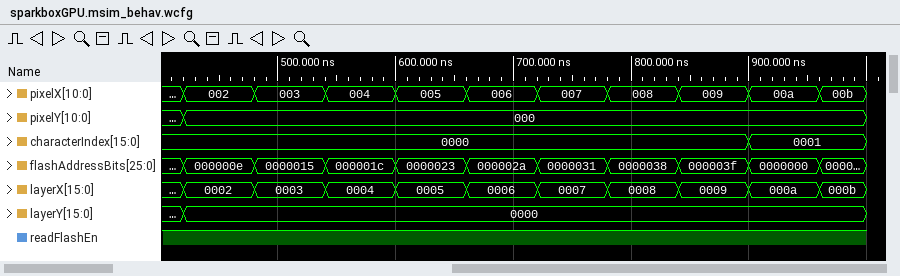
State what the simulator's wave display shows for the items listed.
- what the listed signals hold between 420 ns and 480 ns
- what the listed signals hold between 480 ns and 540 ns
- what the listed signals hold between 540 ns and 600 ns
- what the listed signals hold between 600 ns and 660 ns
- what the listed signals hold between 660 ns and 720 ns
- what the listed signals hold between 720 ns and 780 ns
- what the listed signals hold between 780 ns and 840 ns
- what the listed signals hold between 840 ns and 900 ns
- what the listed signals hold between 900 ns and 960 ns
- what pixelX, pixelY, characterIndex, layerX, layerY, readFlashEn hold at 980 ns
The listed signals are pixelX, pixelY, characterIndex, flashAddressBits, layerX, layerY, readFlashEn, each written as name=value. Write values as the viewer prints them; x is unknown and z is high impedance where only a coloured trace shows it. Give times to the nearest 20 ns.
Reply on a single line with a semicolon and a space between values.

pixelX=002, pixelY=000, characterIndex=0000, flashAddressBits=000000e, layerX=0002, layerY=0000, readFlashEn=1; pixelX=003, pixelY=000, characterIndex=0000, flashAddressBits=0000015, layerX=0003, layerY=0000, readFlashEn=1; pixelX=004, pixelY=000, characterIndex=0000, flashAddressBits=000001c, layerX=0004, layerY=0000, readFlashEn=1; pixelX=005, pixelY=000, characterIndex=0000, flashAddressBits=0000023, layerX=0005, layerY=0000, readFlashEn=1; pixelX=006, pixelY=000, characterIndex=0000, flashAddressBits=000002a, layerX=0006, layerY=0000, readFlashEn=1; pixelX=007, pixelY=000, characterIndex=0000, flashAddressBits=0000031, layerX=0007, layerY=0000, readFlashEn=1; pixelX=008, pixelY=000, characterIndex=0000, flashAddressBits=0000038, layerX=0008, layerY=0000, readFlashEn=1; pixelX=009, pixelY=000, characterIndex=0000, flashAddressBits=000003f, layerX=0009, layerY=0000, readFlashEn=1; pixelX=00a, pixelY=000, characterIndex=0001, flashAddressBits=0000000, layerX=000a, layerY=0000, readFlashEn=1; pixelX=00b, pixelY=000, characterIndex=0001, layerX=000b, layerY=0000, readFlashEn=1
